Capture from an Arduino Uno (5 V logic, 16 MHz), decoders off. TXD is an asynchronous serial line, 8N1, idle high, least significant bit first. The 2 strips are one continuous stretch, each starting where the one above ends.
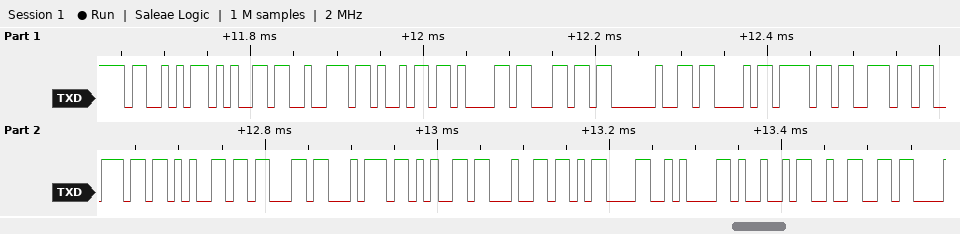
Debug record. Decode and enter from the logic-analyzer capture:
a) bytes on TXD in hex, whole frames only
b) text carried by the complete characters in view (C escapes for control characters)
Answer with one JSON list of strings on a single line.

["0x53 0x65 0x72 0x69 0x61 0x6C 0x20 0x43 0x6F 0x6E 0x6E 0x65 0x63 0x74 0x65 0x64 0x0D 0x0A 0x49 0x32", "\"Serial Connected\\r\\nI2\""]
